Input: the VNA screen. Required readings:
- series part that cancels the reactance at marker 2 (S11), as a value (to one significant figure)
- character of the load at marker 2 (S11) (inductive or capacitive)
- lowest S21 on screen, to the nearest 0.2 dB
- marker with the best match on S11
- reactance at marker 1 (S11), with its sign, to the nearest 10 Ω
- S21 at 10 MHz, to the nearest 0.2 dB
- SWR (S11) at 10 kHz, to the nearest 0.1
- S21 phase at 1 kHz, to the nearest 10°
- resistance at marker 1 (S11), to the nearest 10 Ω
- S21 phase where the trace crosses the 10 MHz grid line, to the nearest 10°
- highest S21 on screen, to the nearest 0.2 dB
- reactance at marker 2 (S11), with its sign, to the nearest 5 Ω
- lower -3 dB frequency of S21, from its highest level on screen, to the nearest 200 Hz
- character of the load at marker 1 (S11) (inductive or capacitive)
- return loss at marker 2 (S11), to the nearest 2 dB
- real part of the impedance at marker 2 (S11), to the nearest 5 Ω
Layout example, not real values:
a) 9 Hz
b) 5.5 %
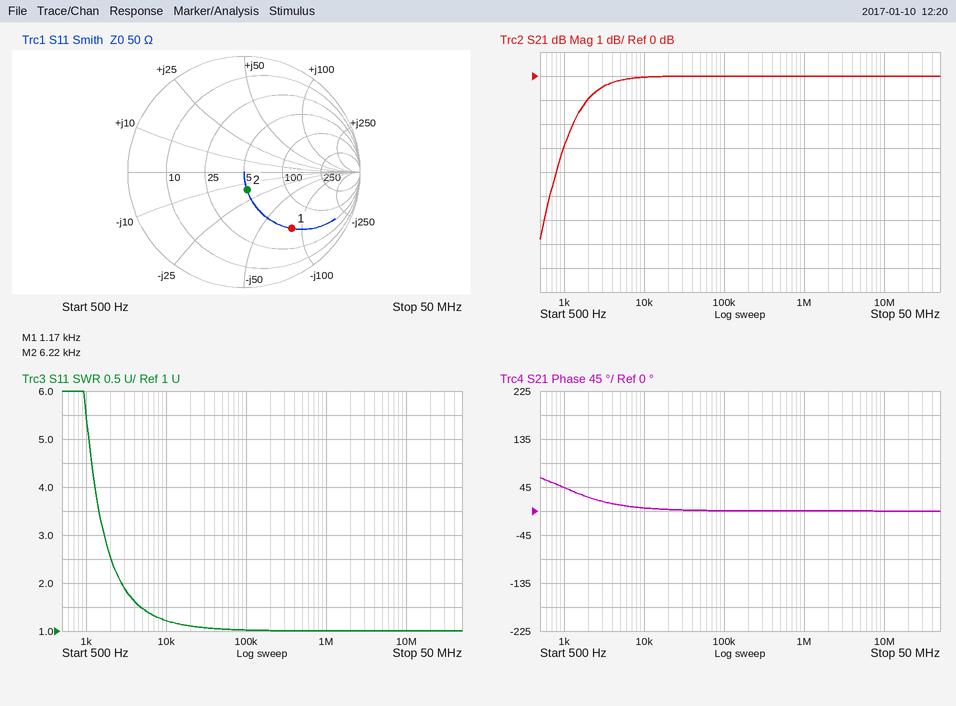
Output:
a) 400 µH
b) capacitive
c) -6.8 dB
d) marker 2
e) -80 Ω
f) 0.0 dB
g) 1.2
h) 40°
i) 50 Ω
j) 0°
k) 0.0 dB
l) -15 Ω
m) 1.0 kHz
n) capacitive
o) 16 dB
p) 50 Ω
